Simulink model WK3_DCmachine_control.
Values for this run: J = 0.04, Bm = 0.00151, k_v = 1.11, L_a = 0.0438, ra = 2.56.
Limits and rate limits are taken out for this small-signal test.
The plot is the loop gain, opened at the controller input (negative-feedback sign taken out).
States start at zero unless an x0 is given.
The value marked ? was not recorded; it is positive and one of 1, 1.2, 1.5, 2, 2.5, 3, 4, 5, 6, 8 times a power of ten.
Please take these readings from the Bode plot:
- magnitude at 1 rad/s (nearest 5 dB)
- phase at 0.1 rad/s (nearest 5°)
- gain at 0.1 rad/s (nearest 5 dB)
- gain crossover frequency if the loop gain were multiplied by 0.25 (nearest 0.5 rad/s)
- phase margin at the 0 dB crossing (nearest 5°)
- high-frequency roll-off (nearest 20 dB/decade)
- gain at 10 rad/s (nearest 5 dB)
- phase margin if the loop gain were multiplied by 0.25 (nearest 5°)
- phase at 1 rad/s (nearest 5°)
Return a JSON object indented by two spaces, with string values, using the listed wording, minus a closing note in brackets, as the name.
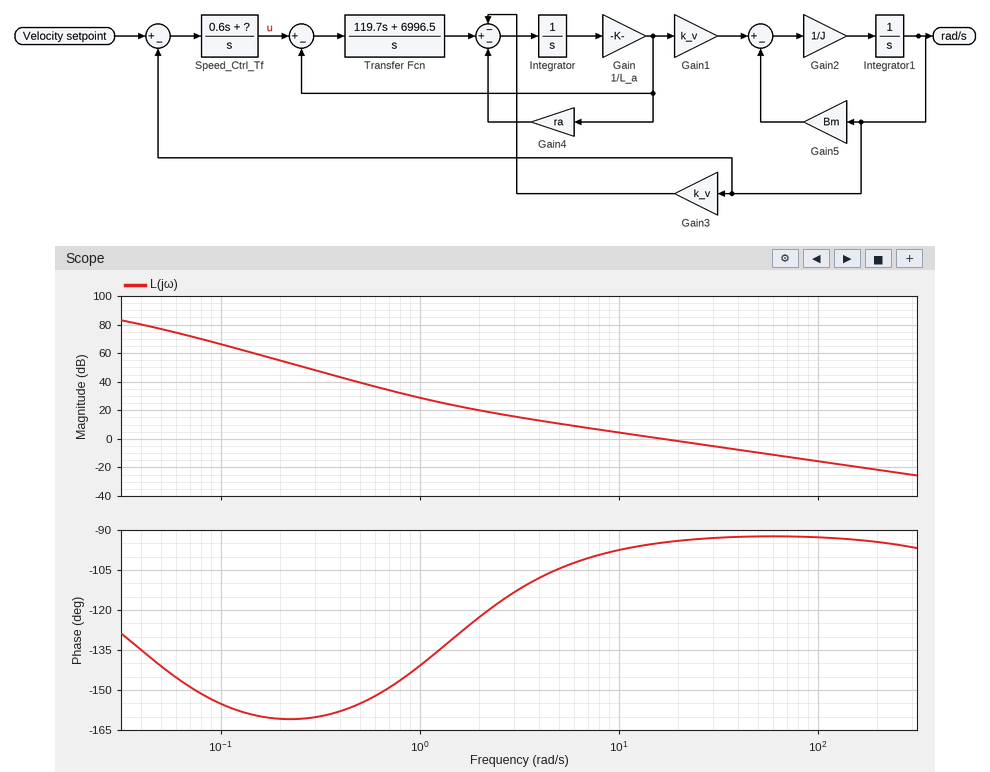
{
  "magnitude at 1 rad/s": "30 dB",
  "phase at 0.1 rad/s": "-155°",
  "gain at 0.1 rad/s": "65 dB",
  "gain crossover frequency if the loop gain were multiplied by 0.25": "4.5 rad/s",
  "phase margin at the 0 dB crossing": "85°",
  "high-frequency roll-off": "-20 dB/decade",
  "gain at 10 rad/s": "5 dB",
  "phase margin if the loop gain were multiplied by 0.25": "75°",
  "phase at 1 rad/s": "-140°"
}
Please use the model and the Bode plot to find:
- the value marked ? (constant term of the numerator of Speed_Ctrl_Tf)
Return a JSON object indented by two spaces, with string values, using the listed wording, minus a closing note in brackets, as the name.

{
  "the value marked ?": "0.8"
}
